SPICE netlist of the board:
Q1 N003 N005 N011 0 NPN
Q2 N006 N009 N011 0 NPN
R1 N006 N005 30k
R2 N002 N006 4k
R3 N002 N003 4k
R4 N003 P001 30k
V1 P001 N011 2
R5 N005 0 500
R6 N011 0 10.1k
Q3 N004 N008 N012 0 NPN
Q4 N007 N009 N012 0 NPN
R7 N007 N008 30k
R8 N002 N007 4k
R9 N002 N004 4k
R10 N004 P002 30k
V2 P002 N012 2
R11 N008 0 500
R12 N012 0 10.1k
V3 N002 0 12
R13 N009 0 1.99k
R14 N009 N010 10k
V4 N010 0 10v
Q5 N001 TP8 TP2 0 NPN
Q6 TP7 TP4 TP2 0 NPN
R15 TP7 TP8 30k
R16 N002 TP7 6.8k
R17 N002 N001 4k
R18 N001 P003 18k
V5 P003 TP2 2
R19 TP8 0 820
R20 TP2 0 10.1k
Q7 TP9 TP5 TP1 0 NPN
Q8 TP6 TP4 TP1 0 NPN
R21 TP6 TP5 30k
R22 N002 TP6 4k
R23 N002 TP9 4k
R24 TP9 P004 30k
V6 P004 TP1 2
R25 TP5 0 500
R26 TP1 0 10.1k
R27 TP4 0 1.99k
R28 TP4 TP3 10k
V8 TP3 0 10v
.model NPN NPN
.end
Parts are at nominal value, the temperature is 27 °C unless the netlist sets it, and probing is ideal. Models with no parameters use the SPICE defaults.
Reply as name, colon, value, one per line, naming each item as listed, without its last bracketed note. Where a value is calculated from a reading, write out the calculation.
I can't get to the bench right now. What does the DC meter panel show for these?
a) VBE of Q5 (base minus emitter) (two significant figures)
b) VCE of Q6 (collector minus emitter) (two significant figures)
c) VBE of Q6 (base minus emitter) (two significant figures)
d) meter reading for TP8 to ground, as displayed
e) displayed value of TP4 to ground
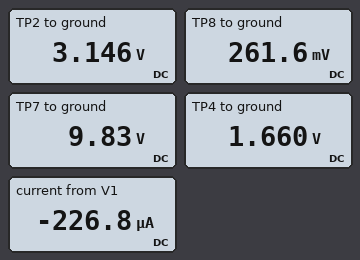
VBE of Q5 (base minus emitter): 261.6 mV - 3.146 V = -2.9 V
VCE of Q6 (collector minus emitter): 9.83 V - 3.146 V = 6.7 V
VBE of Q6 (base minus emitter): 1.66 V - 3.146 V = -1.5 V
meter reading for TP8 to ground, as displayed: 261.6 mV
displayed value of TP4 to ground: 1.660 V
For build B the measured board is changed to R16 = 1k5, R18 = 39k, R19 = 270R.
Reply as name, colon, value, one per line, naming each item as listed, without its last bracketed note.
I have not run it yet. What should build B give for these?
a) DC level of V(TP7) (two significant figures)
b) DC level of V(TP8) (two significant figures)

DC level of V(TP7): 11 V
DC level of V(TP8): 100 mV
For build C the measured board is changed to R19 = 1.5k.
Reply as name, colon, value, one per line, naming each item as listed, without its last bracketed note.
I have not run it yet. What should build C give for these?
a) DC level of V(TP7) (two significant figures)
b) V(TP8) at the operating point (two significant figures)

DC level of V(TP7): 9.9 V
V(TP8) at the operating point: 470 mV
